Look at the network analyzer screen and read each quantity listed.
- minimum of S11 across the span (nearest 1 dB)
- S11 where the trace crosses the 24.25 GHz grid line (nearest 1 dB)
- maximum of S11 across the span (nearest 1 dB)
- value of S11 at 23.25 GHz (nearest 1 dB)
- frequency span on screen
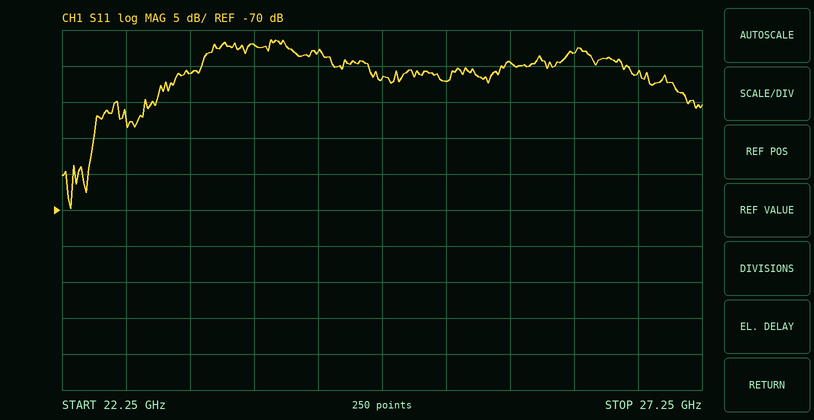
-70 dB
-48 dB
-46 dB
-51 dB
5 GHz
